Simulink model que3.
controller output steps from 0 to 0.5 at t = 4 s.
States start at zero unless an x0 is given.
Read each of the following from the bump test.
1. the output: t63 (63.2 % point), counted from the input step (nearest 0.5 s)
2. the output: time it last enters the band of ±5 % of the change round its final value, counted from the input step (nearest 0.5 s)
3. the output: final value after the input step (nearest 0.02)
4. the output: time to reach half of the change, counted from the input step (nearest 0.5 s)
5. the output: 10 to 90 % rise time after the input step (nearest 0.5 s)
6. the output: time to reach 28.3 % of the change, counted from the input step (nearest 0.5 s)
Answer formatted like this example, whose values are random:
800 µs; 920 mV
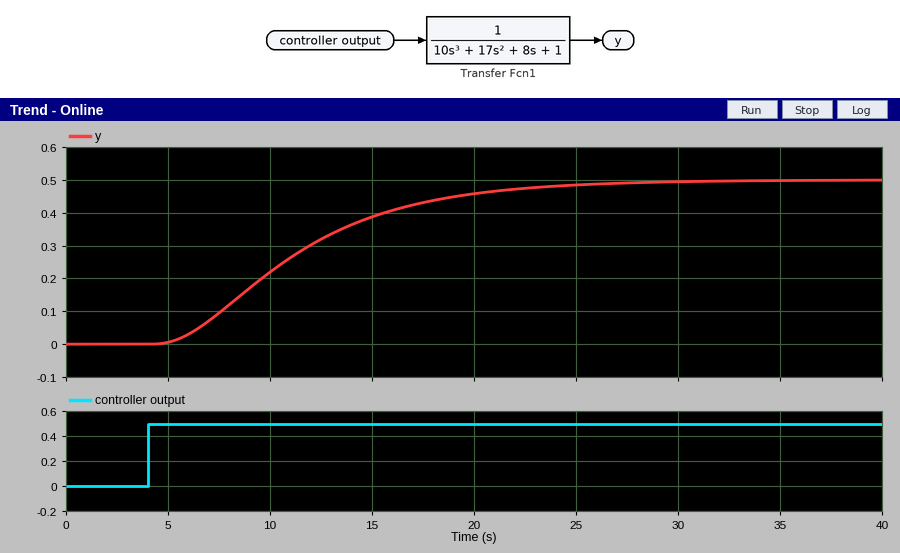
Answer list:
8.5 s; 18.5 s; 0.50; 6.5 s; 12.5 s; 4.5 s
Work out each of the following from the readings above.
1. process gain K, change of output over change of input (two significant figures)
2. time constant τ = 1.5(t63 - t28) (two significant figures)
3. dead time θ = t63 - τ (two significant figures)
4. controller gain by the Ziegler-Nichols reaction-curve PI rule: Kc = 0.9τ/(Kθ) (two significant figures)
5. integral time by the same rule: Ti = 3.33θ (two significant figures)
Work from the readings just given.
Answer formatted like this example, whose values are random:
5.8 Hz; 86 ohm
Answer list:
1.0; 6.0 s; 2.5 s; 2.2; 8.3 s
